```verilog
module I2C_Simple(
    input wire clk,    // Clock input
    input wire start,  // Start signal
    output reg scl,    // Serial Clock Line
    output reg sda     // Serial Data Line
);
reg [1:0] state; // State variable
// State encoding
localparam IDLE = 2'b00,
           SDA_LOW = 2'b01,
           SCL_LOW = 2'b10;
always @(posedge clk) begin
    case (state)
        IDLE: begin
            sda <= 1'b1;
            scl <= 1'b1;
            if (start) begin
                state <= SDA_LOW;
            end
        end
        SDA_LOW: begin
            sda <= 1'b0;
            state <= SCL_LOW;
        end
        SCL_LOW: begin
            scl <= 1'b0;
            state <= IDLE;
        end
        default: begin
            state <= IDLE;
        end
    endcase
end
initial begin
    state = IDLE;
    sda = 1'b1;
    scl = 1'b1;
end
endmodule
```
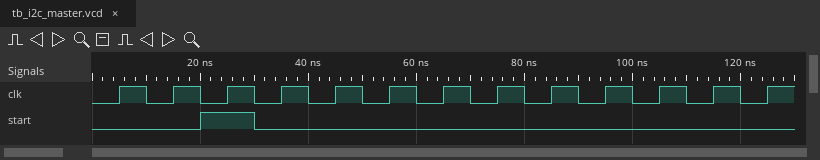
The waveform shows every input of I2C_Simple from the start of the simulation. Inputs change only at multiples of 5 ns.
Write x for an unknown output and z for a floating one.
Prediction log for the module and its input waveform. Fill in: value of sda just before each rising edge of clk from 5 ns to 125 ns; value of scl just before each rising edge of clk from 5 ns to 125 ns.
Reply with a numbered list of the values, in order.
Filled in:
1. 1 1 1 1 0 0 1 1 1 1 1 1 1
2. 1 1 1 1 1 0 1 1 1 1 1 1 1
